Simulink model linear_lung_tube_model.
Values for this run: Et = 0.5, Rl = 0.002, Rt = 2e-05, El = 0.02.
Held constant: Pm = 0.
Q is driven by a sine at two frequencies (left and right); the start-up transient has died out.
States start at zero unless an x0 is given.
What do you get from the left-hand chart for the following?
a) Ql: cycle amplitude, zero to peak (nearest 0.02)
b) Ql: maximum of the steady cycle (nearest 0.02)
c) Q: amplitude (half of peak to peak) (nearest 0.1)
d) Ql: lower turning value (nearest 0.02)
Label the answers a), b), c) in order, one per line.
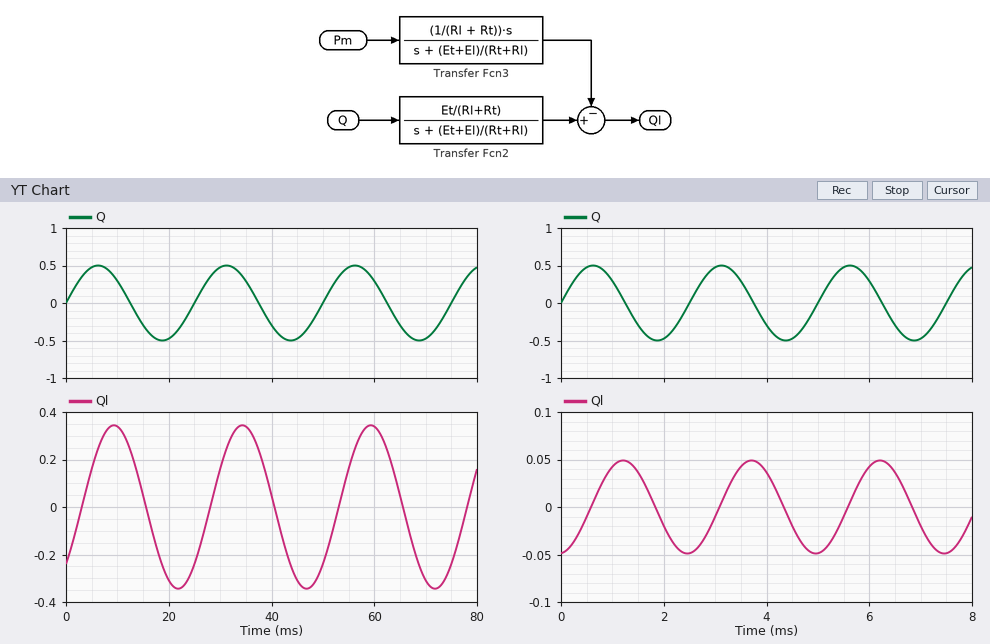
a) 0.34
b) 0.34
c) 0.5
d) -0.34
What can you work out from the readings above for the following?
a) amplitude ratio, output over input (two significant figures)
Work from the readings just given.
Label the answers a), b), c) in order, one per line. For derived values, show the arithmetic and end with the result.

a) 0.34 / 0.5 = 0.68
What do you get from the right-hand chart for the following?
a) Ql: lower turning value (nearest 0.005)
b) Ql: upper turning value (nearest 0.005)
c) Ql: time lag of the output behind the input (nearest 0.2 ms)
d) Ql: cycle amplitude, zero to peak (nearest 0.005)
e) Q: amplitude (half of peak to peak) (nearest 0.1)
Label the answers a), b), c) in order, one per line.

a) -0.050
b) 0.050
c) 0.6 ms
d) 0.050
e) 0.5
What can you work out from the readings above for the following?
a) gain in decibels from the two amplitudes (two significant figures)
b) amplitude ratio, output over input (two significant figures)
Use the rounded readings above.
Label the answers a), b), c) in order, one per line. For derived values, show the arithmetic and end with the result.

a) 20 log10(0.05 / 0.5) = -20 dB
b) 0.05 / 0.5 = 0.10
